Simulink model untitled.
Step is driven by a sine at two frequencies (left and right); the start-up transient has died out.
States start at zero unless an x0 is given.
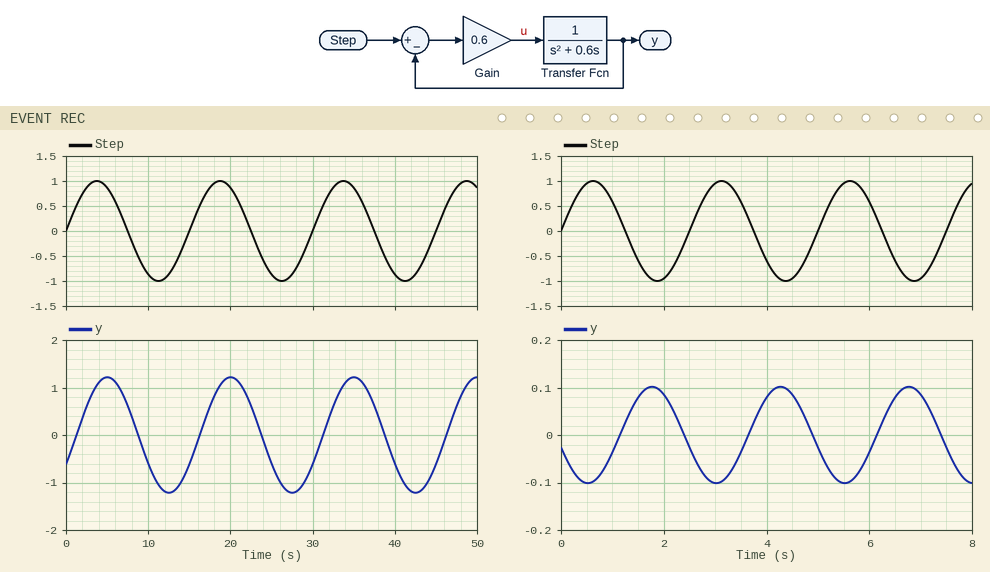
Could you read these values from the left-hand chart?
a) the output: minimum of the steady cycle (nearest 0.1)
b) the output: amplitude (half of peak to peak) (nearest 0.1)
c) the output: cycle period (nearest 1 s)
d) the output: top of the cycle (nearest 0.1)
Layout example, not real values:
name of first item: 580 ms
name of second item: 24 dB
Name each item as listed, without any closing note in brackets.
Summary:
the output: minimum of the steady cycle: -1.2
the output: amplitude (half of peak to peak): 1.2
the output: cycle period: 15 s
the output: top of the cycle: 1.2
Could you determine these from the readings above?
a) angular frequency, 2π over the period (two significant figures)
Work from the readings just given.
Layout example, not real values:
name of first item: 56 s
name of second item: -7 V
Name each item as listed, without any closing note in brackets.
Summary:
angular frequency, 2π over the period: 0.42 rad/s
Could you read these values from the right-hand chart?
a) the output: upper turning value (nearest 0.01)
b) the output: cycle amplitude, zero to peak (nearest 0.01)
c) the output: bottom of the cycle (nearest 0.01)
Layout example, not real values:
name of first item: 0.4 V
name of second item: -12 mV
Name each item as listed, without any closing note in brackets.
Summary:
the output: upper turning value: 0.10
the output: cycle amplitude, zero to peak: 0.10
the output: bottom of the cycle: -0.10
